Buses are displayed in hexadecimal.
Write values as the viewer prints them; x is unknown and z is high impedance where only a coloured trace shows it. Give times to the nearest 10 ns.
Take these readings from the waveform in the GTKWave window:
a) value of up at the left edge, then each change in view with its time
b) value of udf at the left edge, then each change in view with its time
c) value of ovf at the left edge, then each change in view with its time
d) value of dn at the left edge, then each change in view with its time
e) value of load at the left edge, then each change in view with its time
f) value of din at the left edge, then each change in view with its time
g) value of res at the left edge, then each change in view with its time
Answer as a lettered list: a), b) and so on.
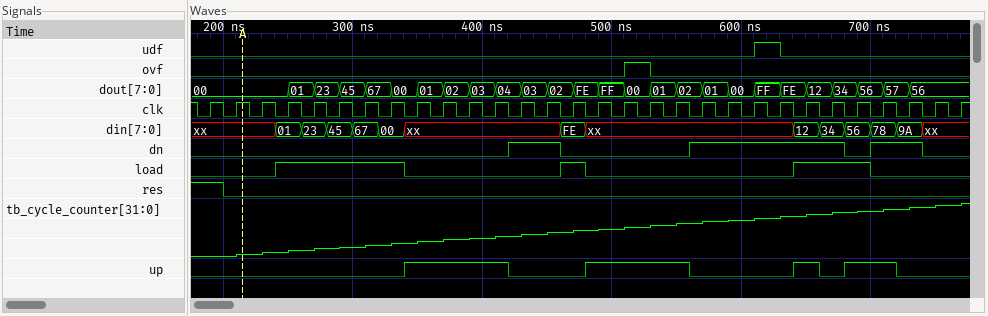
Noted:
a) 0, 1 at 340 ns, 0 at 420 ns, 1 at 480 ns, 0 at 560 ns, 1 at 640 ns, 0 at 660 ns, 1 at 680 ns, 0 at 720 ns
b) 0, 1 at 610 ns, 0 at 630 ns
c) 0, 1 at 510 ns, 0 at 530 ns
d) 0, 1 at 420 ns, 0 at 460 ns, 1 at 560 ns, 0 at 680 ns, 1 at 700 ns, 0 at 740 ns
e) 0, 1 at 240 ns, 0 at 340 ns, 1 at 460 ns, 0 at 480 ns, 1 at 640 ns, 0 at 700 ns
f) xx, 01 at 240 ns, 23 at 260 ns, 45 at 280 ns, 67 at 300 ns, 00 at 320 ns, xx at 340 ns, FE at 460 ns, xx at 480 ns, 12 at 640 ns, 34 at 660 ns, 56 at 680 ns, 78 at 700 ns, 9A at 720 ns, xx at 740 ns
g) 1, 0 at 200 ns
